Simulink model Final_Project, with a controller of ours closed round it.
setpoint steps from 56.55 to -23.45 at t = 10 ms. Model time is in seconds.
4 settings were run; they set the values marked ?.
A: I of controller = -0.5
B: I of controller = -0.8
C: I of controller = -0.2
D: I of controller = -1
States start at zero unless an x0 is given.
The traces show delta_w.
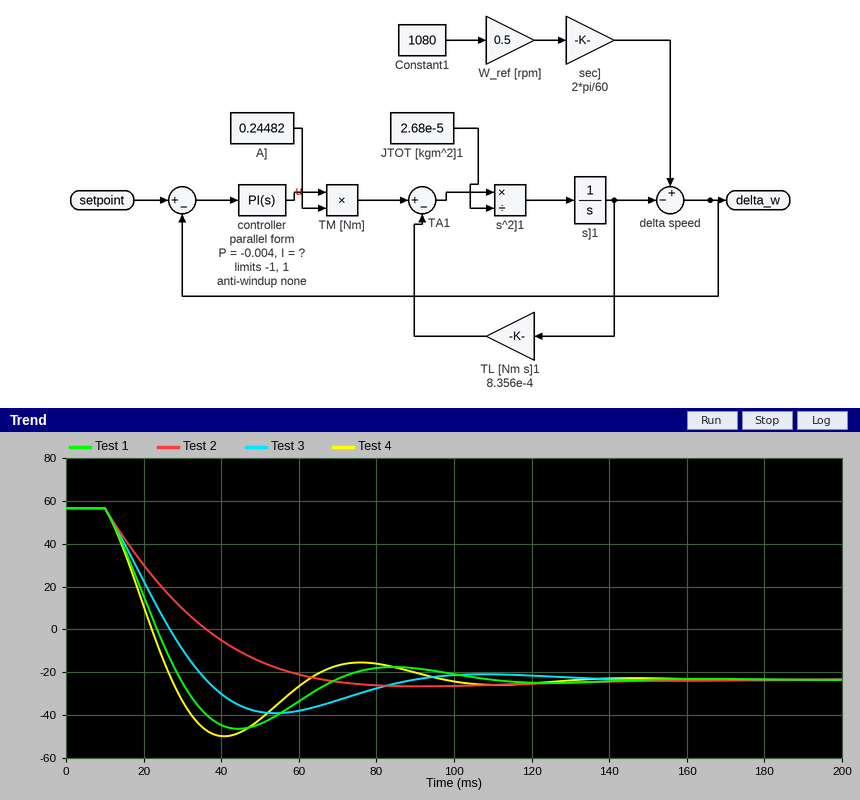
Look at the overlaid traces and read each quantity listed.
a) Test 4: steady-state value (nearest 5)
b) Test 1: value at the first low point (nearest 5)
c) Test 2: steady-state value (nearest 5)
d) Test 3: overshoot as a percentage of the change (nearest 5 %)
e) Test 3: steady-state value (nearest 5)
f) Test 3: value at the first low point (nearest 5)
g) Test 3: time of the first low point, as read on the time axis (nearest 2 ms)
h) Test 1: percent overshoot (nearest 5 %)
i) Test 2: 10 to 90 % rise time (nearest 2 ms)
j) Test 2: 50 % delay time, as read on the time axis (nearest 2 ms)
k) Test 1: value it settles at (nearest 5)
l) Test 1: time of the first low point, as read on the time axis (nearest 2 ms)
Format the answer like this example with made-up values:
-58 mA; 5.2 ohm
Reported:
-25; -45; -25; 20 %; -25; -40; 54 ms; 30 %; 38 ms; 26 ms; -25; 44 ms
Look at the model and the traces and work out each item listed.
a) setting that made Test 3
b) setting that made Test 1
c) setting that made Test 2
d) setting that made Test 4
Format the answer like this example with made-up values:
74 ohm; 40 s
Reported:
A; B; C; D
